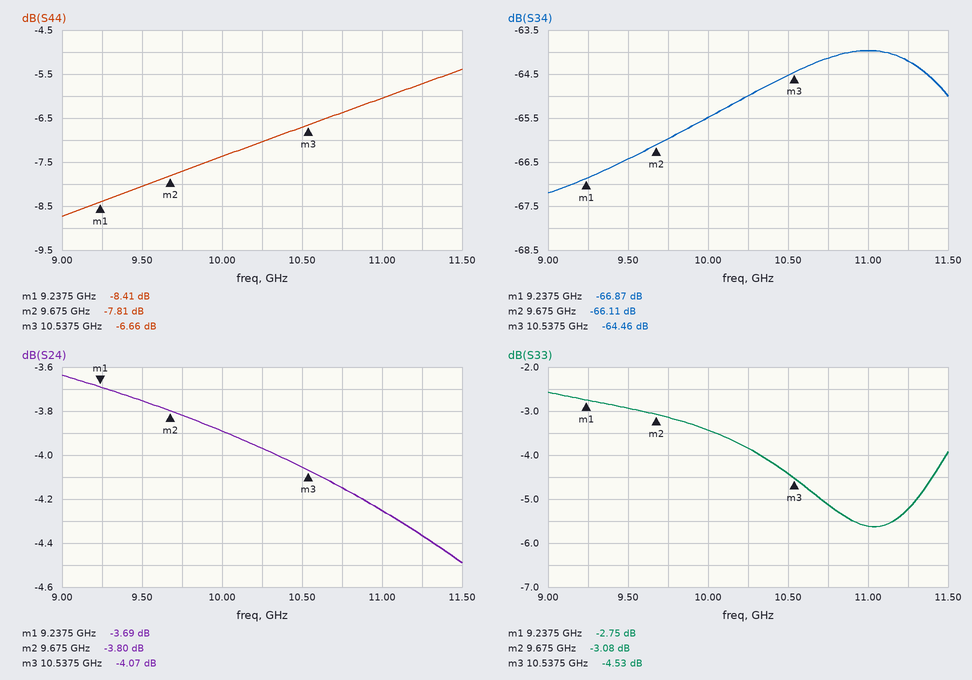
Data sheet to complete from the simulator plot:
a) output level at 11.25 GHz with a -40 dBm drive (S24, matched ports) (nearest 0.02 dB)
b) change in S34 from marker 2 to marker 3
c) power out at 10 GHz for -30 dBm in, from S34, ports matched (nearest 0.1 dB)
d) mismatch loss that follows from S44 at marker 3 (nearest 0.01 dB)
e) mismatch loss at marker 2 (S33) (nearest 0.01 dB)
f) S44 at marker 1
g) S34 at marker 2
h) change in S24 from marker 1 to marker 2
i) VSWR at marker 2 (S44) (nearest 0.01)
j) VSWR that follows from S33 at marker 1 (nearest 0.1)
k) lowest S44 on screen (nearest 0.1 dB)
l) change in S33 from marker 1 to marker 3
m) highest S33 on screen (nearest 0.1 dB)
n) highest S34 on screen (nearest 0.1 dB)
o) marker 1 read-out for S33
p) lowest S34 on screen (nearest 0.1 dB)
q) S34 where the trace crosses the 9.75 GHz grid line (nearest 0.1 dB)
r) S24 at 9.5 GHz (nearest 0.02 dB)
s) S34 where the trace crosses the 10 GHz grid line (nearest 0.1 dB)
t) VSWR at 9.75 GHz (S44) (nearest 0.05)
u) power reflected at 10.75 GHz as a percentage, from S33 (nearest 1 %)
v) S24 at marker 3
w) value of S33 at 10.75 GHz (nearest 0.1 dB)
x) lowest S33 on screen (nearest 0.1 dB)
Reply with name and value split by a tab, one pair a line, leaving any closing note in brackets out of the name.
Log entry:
output level at 11.25 GHz with a -40 dBm drive (S24, matched ports)	-44.36 dBm
change in S34 from marker 2 to marker 3	1.65 dB
power out at 10 GHz for -30 dBm in, from S34, ports matched	-95.5 dBm
mismatch loss that follows from S44 at marker 3	1.06 dB
mismatch loss at marker 2 (S33)	2.94 dB
S44 at marker 1	-8.41 dB
S34 at marker 2	-66.11 dB
change in S24 from marker 1 to marker 2	-0.11 dB
VSWR at marker 2 (S44)	2.37
VSWR that follows from S33 at marker 1	6.4
lowest S44 on screen	-8.7 dB
change in S33 from marker 1 to marker 3	-1.78 dB
highest S33 on screen	-2.6 dB
highest S34 on screen	-64.0 dB
marker 1 read-out for S33	-2.75 dB
lowest S34 on screen	-67.2 dB
S34 where the trace crosses the 9.75 GHz grid line	-66.0 dB
S24 at 9.5 GHz	-3.76 dB
S34 where the trace crosses the 10 GHz grid line	-65.5 dB
VSWR at 9.75 GHz (S44)	2.40
power reflected at 10.75 GHz as a percentage, from S33	31 %
S24 at marker 3	-4.07 dB
value of S33 at 10.75 GHz	-5.1 dB
lowest S33 on screen	-5.6 dB
